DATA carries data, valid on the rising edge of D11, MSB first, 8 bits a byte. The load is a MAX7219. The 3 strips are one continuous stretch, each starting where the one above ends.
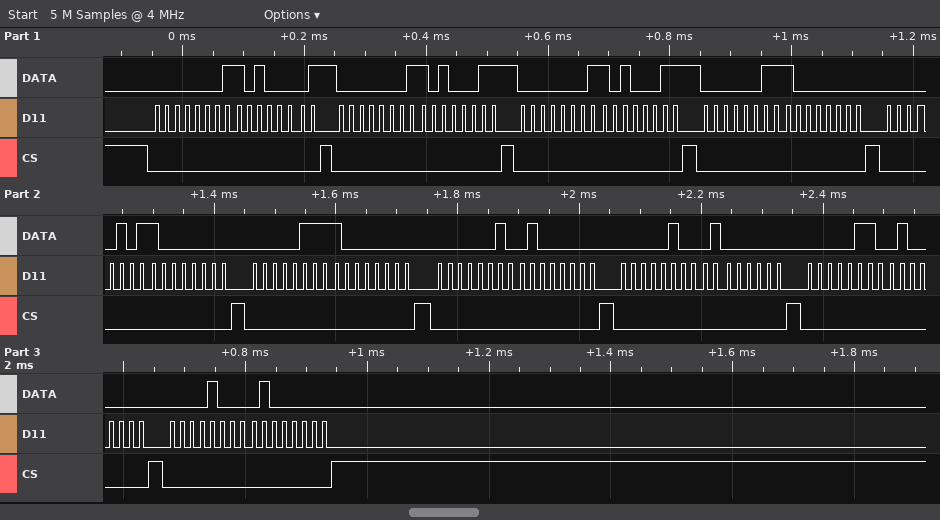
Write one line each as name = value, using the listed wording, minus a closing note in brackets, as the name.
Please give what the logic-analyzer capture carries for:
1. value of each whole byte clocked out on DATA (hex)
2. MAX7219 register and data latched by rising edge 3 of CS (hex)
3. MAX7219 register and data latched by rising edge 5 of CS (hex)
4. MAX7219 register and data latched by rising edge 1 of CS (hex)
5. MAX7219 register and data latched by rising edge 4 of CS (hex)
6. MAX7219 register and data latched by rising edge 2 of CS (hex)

value of each whole byte clocked out on DATA = 01 A1 01 A3 01 A3 03 80 05 80 07 80 02 40 04 40 06 40 08 40
MAX7219 register and data latched by rising edge 3 of CS = register 0x1, data 0xA3
MAX7219 register and data latched by rising edge 5 of CS = register 0x5, data 0x80
MAX7219 register and data latched by rising edge 1 of CS = register 0x1, data 0xA1
MAX7219 register and data latched by rising edge 4 of CS = register 0x3, data 0x80
MAX7219 register and data latched by rising edge 2 of CS = register 0x1, data 0xA3
